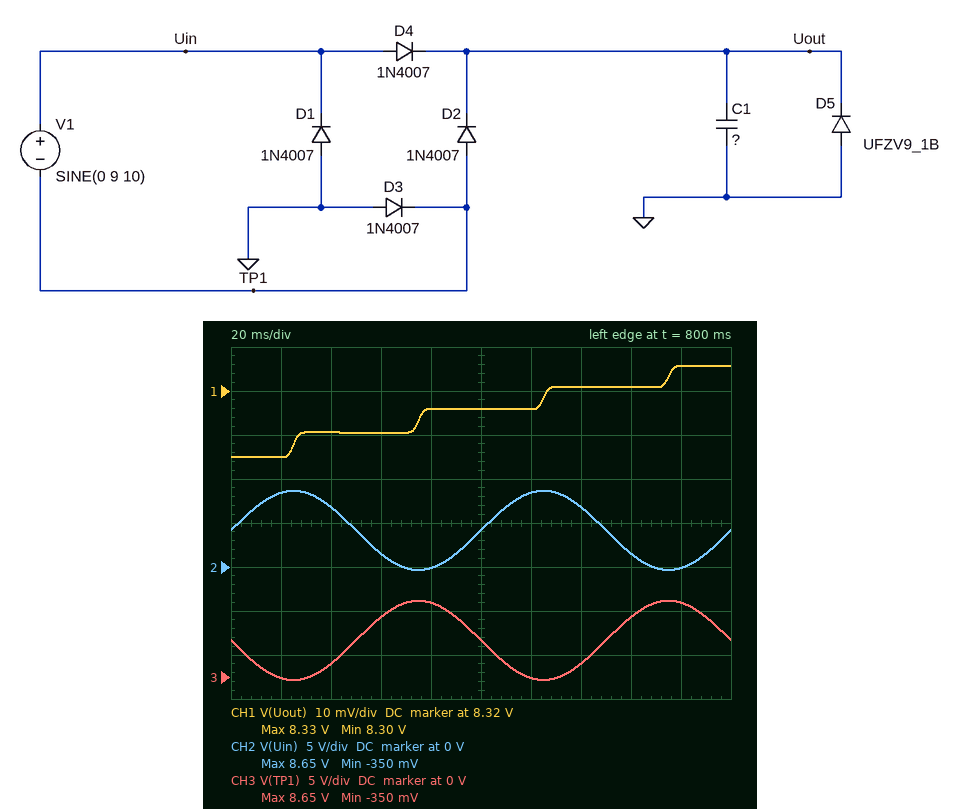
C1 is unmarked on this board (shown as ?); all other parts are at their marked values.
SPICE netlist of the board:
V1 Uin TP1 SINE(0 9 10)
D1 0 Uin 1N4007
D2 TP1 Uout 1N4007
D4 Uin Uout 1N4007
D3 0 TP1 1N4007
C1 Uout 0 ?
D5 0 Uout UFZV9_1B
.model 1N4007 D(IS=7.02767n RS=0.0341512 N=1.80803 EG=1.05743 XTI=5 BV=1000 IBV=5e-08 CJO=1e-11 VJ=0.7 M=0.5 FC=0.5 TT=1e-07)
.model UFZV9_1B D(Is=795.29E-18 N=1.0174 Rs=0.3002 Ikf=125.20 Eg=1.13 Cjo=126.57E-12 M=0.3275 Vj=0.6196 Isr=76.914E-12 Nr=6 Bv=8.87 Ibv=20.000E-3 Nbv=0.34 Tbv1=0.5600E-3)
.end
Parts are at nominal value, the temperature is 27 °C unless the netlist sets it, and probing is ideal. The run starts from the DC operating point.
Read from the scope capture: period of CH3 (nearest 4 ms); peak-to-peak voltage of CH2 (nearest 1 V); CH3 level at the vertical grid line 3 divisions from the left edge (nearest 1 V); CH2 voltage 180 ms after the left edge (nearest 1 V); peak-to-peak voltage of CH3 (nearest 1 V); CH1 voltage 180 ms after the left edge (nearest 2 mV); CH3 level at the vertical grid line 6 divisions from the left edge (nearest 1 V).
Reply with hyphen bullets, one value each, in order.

- 100 ms
- 9 V
- 7 V
- 0 V
- 9 V
- 8.326 V
- 0 V
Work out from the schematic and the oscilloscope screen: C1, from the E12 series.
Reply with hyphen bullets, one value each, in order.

- 8.2 µF
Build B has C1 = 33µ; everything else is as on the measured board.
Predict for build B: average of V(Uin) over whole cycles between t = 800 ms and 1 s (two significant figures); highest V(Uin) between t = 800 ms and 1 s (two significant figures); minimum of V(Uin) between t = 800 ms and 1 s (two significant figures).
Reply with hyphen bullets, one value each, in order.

- 4.1 V
- 8.6 V
- -410 mV
